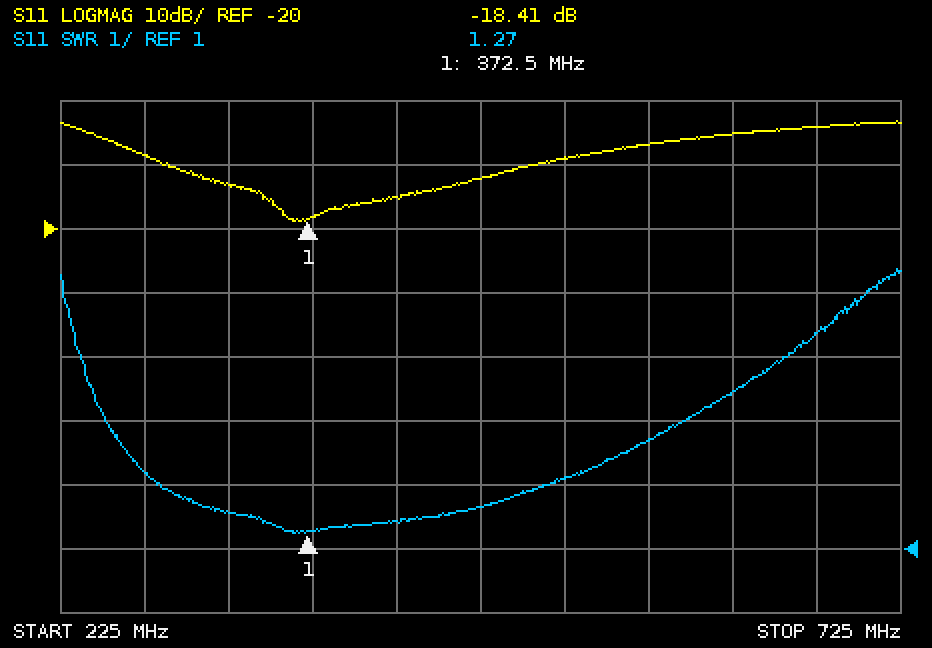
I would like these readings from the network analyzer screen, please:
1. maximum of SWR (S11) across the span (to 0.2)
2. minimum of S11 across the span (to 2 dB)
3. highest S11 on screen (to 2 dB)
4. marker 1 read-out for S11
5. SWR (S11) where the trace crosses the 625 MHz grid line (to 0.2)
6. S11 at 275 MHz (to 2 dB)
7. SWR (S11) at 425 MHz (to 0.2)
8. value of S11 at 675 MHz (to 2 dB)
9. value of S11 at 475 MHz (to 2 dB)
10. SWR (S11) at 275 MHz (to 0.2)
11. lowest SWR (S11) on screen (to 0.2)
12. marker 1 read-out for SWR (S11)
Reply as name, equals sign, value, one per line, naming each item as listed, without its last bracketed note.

maximum of SWR (S11) across the span = 5.4
minimum of S11 across the span = -18 dB
highest S11 on screen = -4 dB
marker 1 read-out for S11 = -18.41 dB
SWR (S11) where the trace crosses the 625 MHz grid line = 3.4
S11 at 275 MHz = -8 dB
SWR (S11) at 425 MHz = 1.4
value of S11 at 675 MHz = -4 dB
value of S11 at 475 MHz = -12 dB
SWR (S11) at 275 MHz = 2.2
lowest SWR (S11) on screen = 1.2
marker 1 read-out for SWR = 1.27
